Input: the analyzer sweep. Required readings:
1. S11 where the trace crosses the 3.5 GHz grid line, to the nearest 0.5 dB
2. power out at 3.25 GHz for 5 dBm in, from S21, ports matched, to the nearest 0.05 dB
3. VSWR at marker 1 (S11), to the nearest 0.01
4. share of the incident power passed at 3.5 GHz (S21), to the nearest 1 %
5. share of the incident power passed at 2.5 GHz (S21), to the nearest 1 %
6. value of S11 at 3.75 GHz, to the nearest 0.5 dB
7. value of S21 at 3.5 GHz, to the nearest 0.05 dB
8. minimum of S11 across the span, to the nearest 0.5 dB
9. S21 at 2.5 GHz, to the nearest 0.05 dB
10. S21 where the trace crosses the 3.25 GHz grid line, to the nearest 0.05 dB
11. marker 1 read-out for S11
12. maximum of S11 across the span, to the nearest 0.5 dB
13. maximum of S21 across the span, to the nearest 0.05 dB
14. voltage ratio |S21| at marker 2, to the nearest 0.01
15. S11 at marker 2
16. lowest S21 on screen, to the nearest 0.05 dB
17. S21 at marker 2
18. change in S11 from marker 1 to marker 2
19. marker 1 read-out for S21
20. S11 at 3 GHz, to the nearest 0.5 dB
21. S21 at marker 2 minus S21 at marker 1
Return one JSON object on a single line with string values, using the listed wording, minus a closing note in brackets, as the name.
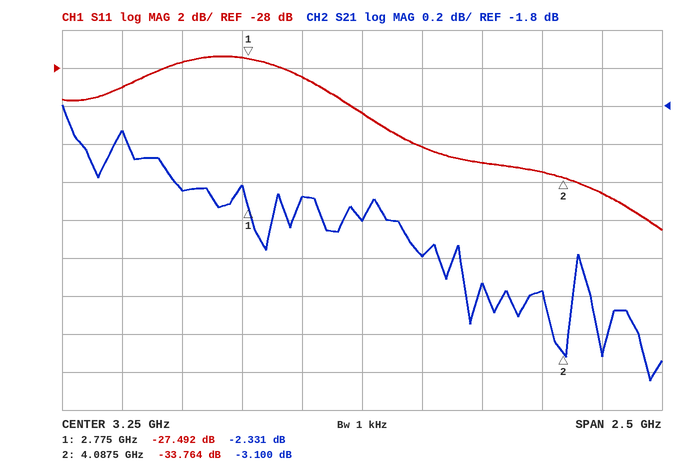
{"S11 where the trace crosses the 3.5 GHz grid line, to the nearest 0.5 dB": "-32.0 dB", "power out at 3.25 GHz for 5 dBm in, from S21, ports matched, to the nearest 0.05 dB": "2.60 dBm", "VSWR at marker 1 (S11), to the nearest 0.01": "1.09", "share of the incident power passed at 3.5 GHz (S21), to the nearest 1 %": "55 %", "share of the incident power passed at 2.5 GHz (S21), to the nearest 1 %": "60 %", "value of S11 at 3.75 GHz, to the nearest 0.5 dB": "-33.0 dB", "value of S21 at 3.5 GHz, to the nearest 0.05 dB": "-2.60 dB", "minimum of S11 across the span, to the nearest 0.5 dB": "-36.5 dB", "S21 at 2.5 GHz, to the nearest 0.05 dB": "-2.25 dB", "S21 where the trace crosses the 3.25 GHz grid line, to the nearest 0.05 dB": "-2.40 dB", "marker 1 read-out for S11": "-27.492 dB", "maximum of S11 across the span, to the nearest 0.5 dB": "-27.5 dB", "maximum of S21 across the span, to the nearest 0.05 dB": "-1.80 dB", "voltage ratio |S21| at marker 2, to the nearest 0.01": "0.70", "S11 at marker 2": "-33.764 dB", "lowest S21 on screen, to the nearest 0.05 dB": "-3.25 dB", "S21 at marker 2": "-3.100 dB", "change in S11 from marker 1 to marker 2": "-6.272 dB", "marker 1 read-out for S21": "-2.331 dB", "S11 at 3 GHz, to the nearest 0.5 dB": "-28.5 dB", "S21 at marker 2 minus S21 at marker 1": "-0.769 dB"}
